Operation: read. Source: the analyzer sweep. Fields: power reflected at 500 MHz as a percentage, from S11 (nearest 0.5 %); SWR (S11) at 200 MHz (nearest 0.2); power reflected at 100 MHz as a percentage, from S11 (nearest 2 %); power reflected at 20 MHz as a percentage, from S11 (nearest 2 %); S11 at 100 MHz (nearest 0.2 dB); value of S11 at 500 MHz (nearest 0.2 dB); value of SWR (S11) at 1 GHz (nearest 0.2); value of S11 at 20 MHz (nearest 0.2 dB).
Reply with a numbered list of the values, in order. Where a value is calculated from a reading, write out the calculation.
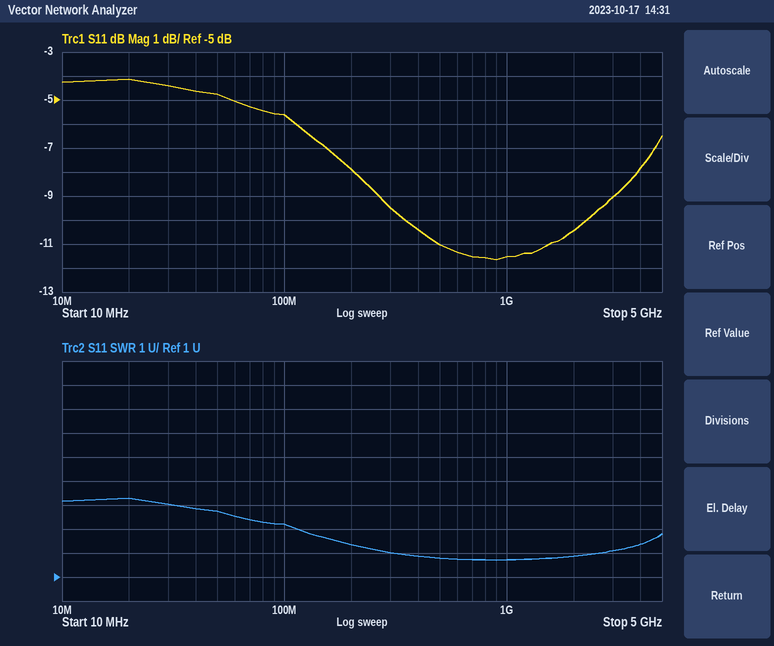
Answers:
1. 10^(-11/10) ≈ 7.94 %, so 8.0 % to the nearest 0.5 %
2. 2.4
3. 10^(-5.6/10) ≈ 28 %
4. 10^(-4.2/10) ≈ 38 %
5. -5.6 dB
6. -11.0 dB
7. 1.8
8. -4.2 dB
